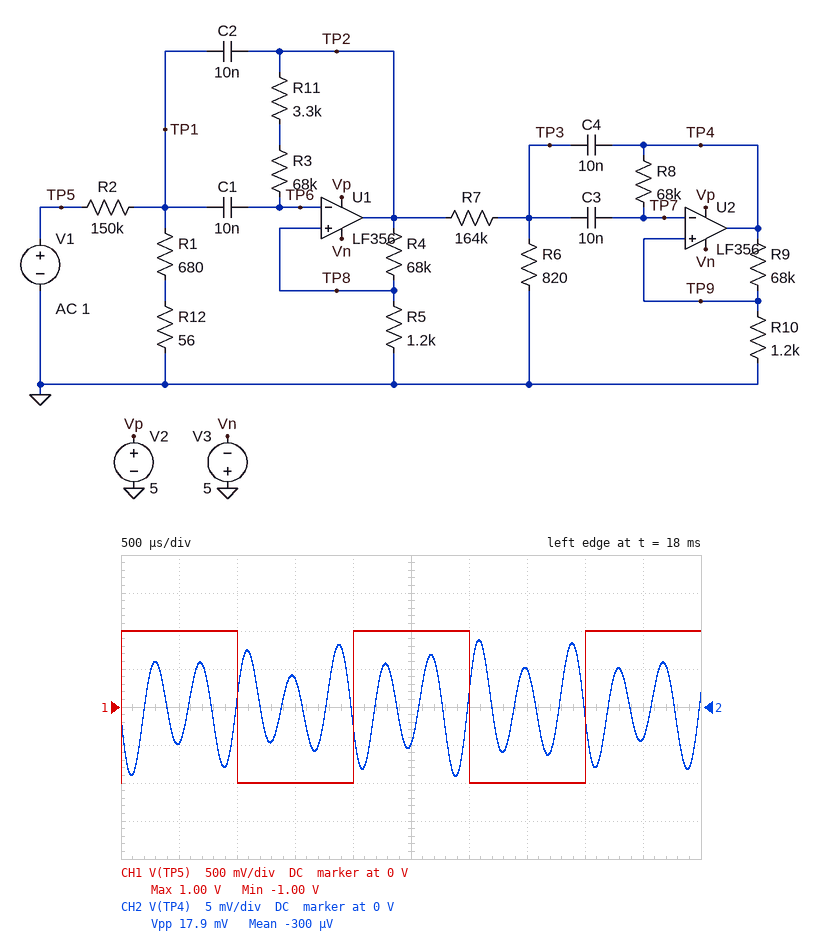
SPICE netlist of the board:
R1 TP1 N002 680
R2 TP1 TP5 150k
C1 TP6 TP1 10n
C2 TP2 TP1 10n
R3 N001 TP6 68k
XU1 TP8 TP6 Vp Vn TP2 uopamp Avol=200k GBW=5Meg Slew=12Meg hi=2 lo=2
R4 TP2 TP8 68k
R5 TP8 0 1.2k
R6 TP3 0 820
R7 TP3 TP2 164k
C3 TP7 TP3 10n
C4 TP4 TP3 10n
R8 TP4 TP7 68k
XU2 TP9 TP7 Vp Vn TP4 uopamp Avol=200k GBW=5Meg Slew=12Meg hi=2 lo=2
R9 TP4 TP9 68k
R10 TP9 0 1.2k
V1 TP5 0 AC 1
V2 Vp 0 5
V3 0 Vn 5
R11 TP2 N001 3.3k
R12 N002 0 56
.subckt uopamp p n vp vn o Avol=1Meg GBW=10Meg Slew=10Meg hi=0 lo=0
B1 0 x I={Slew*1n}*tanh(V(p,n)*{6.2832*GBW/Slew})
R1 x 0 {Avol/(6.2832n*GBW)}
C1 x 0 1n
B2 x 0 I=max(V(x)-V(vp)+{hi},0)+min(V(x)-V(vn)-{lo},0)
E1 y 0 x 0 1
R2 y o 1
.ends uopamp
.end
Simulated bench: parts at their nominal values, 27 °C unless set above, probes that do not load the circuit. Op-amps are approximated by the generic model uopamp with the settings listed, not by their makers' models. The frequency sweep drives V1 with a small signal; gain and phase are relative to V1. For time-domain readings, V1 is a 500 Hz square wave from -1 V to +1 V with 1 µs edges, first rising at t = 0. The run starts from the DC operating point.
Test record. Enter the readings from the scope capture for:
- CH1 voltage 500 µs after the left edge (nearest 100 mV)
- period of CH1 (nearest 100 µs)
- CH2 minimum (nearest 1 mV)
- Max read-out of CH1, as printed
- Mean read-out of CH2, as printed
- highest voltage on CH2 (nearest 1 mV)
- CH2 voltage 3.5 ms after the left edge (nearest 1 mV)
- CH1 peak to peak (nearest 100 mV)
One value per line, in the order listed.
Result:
1.0 V
2.0 ms
-9 mV
1.00 V
-300 µV
9 mV
5 mV
2.0 V
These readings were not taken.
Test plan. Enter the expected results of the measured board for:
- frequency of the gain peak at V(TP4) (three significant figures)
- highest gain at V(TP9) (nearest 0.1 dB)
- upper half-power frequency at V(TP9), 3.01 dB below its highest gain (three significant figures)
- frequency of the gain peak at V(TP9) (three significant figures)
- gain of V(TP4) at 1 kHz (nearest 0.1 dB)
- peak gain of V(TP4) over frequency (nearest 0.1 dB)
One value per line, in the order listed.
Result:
2.19 kHz
-35.4 dB
2.22 kHz
2.19 kHz
-62.2 dB
-0.2 dB
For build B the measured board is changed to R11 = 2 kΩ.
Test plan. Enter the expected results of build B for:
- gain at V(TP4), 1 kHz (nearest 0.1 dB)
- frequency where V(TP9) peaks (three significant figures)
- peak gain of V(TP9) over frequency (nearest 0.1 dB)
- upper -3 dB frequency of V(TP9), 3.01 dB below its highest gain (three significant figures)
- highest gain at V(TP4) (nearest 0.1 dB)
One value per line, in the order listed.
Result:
-62.4 dB
2.21 kHz
-37.8 dB
2.24 kHz
-2.6 dB
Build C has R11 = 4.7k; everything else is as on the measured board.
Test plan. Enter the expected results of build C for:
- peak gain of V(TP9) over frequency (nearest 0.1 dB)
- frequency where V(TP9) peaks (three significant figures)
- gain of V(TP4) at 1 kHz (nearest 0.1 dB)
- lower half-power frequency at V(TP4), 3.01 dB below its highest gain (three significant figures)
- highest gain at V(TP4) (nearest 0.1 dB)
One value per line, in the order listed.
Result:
-32.8 dB
2.17 kHz
-62.0 dB
2.14 kHz
2.4 dB
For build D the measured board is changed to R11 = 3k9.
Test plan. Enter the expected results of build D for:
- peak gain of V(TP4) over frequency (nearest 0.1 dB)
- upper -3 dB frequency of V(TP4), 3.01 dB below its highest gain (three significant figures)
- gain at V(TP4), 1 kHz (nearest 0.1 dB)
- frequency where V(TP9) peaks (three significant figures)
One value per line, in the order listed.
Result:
0.9 dB
2.21 kHz
-62.1 dB
2.18 kHz
